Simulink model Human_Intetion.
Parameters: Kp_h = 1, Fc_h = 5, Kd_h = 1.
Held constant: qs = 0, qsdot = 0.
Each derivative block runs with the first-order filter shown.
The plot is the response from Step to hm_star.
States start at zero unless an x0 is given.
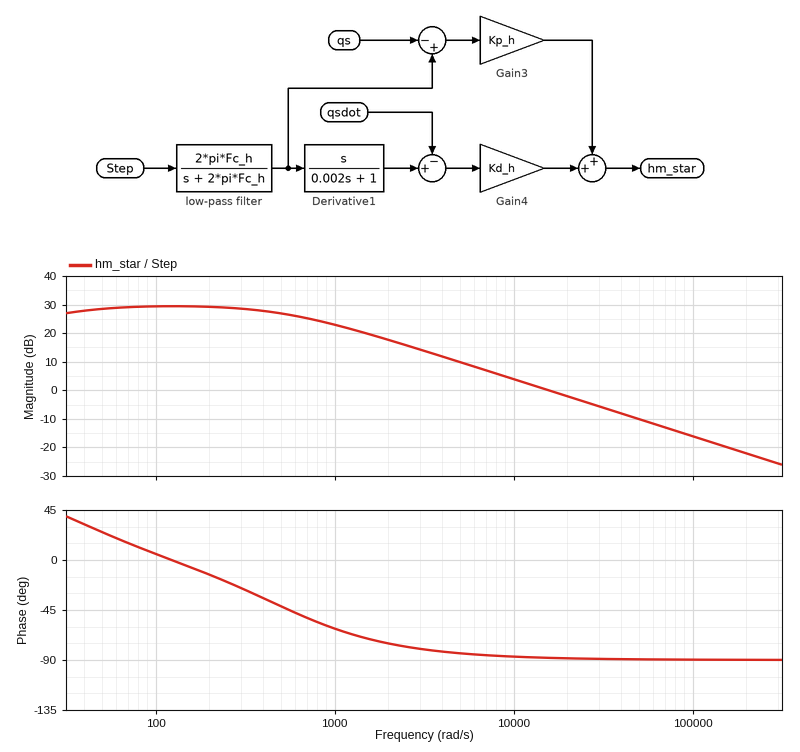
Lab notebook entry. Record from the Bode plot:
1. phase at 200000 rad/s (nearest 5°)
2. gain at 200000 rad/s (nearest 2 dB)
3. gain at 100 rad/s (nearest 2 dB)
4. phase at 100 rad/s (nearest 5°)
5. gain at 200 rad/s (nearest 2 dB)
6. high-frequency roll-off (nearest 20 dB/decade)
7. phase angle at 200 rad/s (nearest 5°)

-90°
-22 dB
30 dB
5°
30 dB
-20 dB/decade
-15°
